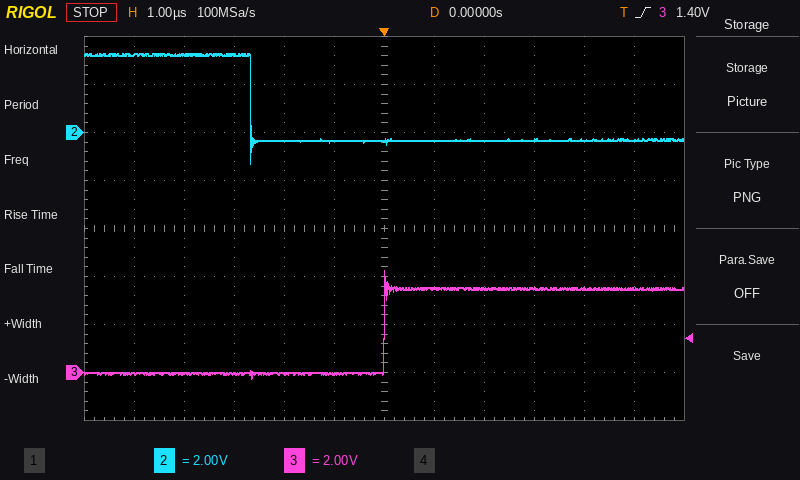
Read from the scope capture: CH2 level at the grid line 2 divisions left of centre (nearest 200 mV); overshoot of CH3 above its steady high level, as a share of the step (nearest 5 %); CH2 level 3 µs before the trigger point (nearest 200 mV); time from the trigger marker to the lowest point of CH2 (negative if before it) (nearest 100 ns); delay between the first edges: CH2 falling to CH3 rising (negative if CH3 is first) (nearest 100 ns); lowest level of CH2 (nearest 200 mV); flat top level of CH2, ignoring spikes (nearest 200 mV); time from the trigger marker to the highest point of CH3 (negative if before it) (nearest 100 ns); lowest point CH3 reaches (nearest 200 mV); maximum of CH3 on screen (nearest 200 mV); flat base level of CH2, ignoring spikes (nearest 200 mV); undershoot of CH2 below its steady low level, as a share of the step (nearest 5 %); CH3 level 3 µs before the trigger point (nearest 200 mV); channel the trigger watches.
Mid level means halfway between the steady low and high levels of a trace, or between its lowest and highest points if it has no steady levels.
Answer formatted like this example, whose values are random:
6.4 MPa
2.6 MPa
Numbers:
-400 mV
20 %
3.2 V
-2.7 µs
+2.7 µs
-1.2 V
3.2 V
0.0 µs
-200 mV
4.2 V
-400 mV
25 %
0.0 V
CH3
